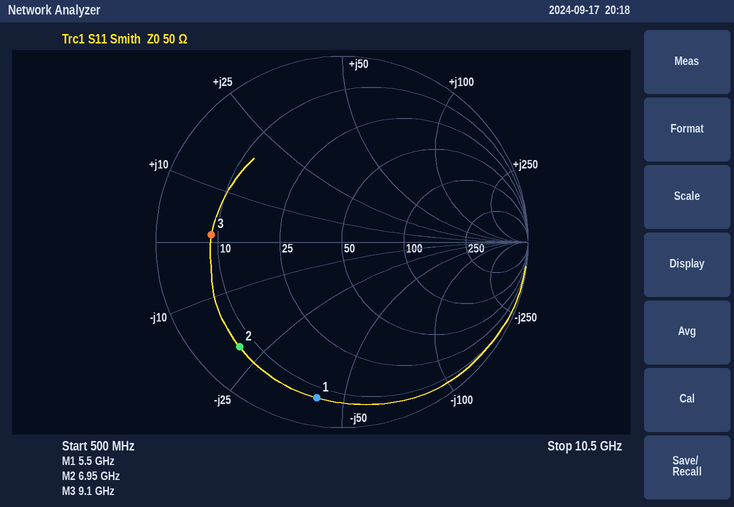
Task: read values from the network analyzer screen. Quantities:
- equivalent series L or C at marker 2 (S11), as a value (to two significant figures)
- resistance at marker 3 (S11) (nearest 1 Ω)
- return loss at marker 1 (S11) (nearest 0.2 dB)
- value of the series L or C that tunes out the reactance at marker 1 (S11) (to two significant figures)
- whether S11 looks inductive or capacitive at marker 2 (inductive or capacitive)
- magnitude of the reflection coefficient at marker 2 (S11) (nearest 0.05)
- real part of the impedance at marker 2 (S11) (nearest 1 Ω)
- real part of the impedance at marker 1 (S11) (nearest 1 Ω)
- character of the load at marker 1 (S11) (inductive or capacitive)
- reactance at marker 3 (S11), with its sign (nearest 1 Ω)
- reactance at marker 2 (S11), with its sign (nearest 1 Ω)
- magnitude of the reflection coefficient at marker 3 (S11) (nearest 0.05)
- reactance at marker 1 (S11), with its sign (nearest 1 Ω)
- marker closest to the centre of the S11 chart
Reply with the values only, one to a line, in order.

1.1 pF
9 Ω
1.4 dB
1.2 nH
capacitive
0.80
7 Ω
7 Ω
capacitive
+1 Ω
-21 Ω
0.70
-42 Ω
marker 3
